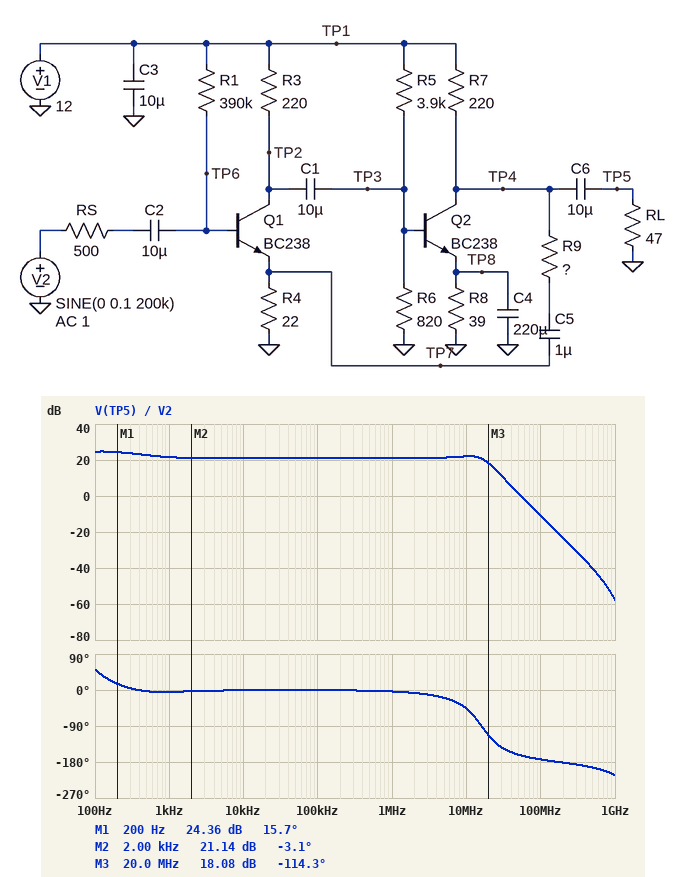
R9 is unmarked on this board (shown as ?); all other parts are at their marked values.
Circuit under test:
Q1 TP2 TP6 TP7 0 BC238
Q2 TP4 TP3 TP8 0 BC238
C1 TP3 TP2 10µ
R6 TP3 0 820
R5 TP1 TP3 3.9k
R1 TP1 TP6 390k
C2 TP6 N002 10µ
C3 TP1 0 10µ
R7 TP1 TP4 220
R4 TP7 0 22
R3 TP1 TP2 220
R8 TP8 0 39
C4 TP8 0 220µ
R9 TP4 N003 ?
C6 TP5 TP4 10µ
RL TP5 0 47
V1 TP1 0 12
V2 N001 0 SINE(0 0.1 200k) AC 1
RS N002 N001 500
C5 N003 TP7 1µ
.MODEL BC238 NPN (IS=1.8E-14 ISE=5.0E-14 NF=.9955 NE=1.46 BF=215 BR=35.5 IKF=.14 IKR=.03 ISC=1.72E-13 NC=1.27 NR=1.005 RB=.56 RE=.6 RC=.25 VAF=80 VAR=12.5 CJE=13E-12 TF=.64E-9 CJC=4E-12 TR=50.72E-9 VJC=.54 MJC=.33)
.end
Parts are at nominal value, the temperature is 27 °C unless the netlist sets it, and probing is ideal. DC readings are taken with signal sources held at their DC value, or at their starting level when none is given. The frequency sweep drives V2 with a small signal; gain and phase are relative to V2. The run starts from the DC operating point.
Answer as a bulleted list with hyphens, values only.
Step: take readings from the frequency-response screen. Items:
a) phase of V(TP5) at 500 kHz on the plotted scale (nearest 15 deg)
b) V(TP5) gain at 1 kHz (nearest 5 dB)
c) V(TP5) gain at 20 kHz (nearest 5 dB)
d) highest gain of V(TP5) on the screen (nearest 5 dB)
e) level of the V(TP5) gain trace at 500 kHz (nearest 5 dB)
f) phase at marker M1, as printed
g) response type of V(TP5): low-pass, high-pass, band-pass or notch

- 0 deg
- 20 dB
- 20 dB
- 25 dB
- 20 dB
- 15.7 deg
- low-pass
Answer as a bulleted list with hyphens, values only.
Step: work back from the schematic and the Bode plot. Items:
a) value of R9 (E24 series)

- 270 Ω
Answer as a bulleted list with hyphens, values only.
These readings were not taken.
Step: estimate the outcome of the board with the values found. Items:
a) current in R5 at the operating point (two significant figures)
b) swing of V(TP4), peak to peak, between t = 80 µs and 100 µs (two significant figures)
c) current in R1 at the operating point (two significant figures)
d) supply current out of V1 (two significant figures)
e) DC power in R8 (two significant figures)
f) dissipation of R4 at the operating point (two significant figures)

- 2.6 mA
- 2.1 V
- 29 µA
- 39 mA
- 37 mW
- 700 µW
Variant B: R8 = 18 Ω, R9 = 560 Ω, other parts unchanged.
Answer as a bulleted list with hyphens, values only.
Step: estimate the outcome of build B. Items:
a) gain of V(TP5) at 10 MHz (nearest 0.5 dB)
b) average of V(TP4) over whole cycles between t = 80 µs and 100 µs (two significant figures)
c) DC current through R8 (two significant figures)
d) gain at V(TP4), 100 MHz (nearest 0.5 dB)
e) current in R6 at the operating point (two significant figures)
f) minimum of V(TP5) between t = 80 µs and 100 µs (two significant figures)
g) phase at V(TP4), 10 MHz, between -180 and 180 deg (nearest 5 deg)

- -22.5 dB
- 1.5 V
- 50 mA
- -47.0 dB
- 2.1 mA
- -140 mV
- -155 deg
